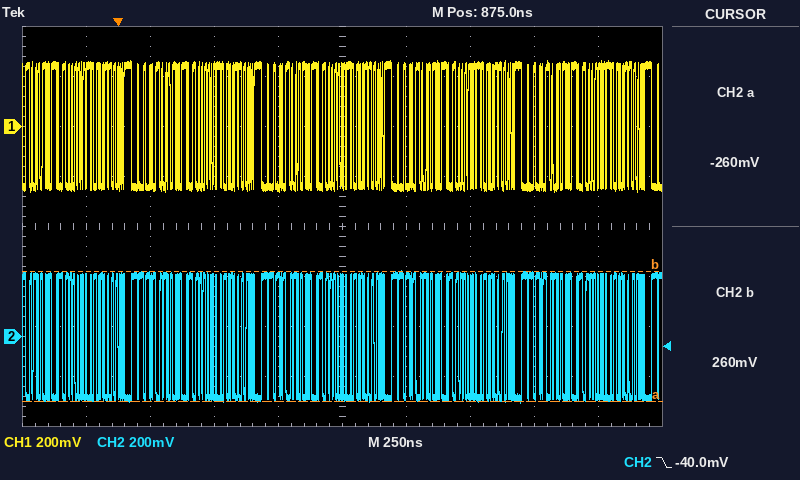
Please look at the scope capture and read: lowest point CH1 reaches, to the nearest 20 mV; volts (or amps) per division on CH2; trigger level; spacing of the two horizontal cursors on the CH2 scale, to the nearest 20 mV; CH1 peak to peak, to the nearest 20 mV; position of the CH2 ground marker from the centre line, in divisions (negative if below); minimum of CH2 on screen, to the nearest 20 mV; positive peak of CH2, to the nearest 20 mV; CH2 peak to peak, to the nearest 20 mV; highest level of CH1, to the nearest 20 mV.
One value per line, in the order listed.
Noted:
-260 mV
200 mV
-40.0 mV
520 mV
520 mV
-2.2 div
-260 mV
260 mV
520 mV
260 mV
